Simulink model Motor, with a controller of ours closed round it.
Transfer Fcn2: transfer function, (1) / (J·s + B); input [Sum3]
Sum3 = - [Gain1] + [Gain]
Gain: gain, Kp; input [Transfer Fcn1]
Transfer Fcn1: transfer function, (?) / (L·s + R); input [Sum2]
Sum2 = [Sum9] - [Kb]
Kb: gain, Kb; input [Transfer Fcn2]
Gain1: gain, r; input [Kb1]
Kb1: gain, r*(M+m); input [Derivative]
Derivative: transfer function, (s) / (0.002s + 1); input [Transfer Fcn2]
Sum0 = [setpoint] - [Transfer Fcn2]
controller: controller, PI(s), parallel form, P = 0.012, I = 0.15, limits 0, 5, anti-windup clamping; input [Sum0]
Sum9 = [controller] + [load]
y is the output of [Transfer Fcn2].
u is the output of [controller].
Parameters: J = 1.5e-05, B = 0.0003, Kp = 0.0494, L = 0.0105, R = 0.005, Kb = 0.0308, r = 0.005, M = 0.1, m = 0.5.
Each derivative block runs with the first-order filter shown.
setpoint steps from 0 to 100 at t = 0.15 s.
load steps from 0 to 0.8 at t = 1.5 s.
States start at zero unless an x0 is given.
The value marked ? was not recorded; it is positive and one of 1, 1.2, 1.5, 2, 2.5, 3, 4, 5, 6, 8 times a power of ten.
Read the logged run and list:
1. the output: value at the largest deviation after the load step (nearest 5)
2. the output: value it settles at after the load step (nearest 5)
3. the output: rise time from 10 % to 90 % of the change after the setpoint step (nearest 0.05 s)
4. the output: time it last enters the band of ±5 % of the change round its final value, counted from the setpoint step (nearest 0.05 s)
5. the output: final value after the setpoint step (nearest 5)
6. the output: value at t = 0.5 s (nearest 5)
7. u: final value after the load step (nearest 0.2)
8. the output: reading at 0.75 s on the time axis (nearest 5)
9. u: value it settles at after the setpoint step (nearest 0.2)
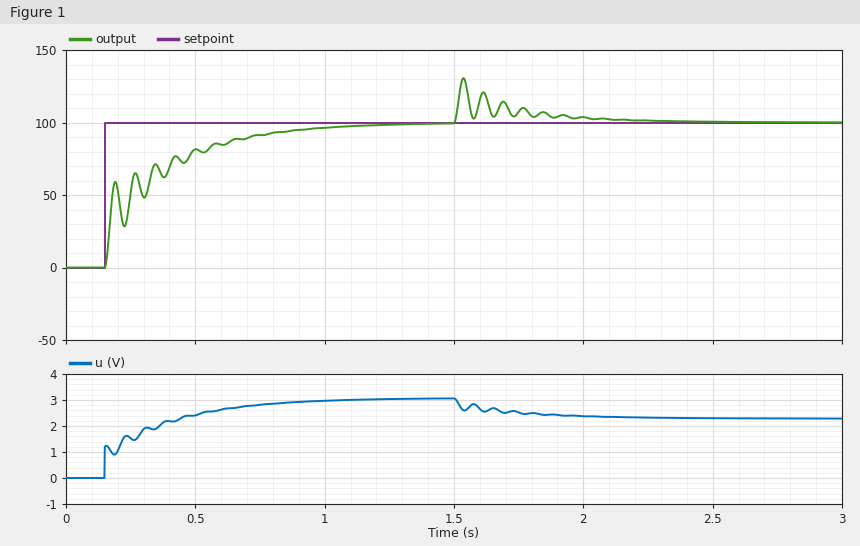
130
100
0.55 s
0.75 s
100
80
2.2
90
3.0
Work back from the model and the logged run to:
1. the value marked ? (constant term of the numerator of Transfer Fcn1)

1
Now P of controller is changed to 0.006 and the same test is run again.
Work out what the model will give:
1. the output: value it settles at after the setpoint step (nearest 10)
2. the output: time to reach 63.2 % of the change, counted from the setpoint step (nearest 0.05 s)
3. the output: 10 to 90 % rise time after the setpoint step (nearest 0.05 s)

100
0.20 s
0.50 s
